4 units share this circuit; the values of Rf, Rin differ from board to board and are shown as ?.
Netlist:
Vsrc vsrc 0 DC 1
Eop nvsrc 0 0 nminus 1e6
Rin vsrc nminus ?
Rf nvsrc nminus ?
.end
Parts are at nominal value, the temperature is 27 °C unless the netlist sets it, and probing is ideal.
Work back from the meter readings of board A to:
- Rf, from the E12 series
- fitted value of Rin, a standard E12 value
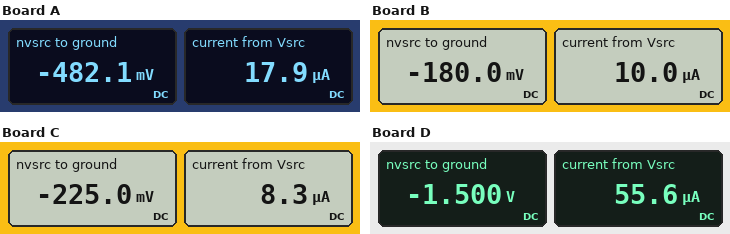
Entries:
27 kΩ
56 kΩ
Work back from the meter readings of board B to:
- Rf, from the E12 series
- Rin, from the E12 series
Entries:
18 kΩ
100 kΩ
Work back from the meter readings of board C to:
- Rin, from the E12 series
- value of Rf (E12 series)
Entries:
120 kΩ
27 kΩ
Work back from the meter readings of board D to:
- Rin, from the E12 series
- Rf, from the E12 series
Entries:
18 kΩ
27 kΩ
